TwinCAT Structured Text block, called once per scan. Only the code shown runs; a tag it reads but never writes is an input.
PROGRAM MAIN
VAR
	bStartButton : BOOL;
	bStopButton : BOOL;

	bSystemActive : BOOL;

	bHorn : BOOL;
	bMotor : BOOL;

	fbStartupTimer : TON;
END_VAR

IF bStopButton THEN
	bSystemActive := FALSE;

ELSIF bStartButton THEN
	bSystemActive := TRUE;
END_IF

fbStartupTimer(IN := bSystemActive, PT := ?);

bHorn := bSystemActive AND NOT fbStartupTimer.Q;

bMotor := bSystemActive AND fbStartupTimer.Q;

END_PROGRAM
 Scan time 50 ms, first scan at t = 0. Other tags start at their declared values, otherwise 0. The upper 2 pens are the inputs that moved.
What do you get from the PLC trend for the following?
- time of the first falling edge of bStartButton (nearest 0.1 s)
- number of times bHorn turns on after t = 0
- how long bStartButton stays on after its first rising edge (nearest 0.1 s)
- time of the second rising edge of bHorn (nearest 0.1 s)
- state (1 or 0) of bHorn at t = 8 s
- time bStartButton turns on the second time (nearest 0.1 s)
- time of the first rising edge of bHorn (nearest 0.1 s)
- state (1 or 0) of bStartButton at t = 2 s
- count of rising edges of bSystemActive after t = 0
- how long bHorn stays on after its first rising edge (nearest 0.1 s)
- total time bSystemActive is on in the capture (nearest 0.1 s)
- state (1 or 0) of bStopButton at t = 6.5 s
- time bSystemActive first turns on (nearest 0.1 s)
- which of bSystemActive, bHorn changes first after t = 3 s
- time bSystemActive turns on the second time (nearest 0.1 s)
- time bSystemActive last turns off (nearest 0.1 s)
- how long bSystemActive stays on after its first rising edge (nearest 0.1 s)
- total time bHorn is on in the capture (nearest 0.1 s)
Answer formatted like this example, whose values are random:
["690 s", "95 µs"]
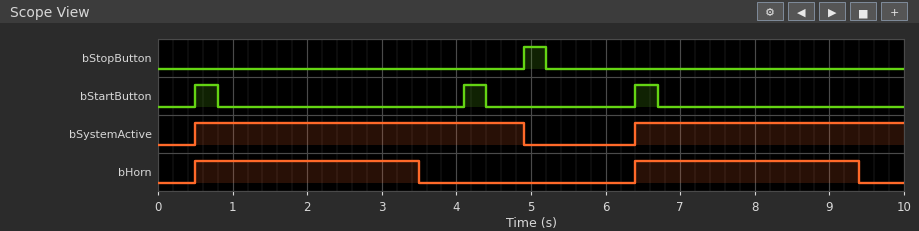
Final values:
["0.8 s", "2", "0.3 s", "6.4 s", "1", "4.1 s", "0.5 s", "0", "2", "3.0 s", "8.0 s", "0", "0.5 s", "bHorn", "6.4 s", "4.9 s", "4.4 s", "6.0 s"]
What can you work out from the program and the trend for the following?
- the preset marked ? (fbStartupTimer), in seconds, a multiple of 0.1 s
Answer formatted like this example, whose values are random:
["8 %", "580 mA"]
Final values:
["3.0 s"]
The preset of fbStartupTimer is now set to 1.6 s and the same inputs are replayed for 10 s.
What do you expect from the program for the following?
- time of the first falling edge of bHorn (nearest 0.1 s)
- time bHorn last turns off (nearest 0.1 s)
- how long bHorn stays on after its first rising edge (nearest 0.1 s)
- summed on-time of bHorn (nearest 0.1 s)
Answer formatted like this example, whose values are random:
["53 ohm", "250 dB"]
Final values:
["2.1 s", "8.0 s", "1.6 s", "3.2 s"]
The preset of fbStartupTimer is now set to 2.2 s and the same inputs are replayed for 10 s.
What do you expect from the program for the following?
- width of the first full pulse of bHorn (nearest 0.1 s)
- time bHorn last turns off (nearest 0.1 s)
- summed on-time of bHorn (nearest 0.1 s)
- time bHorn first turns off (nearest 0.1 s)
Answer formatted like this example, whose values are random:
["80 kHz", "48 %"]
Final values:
["2.2 s", "8.6 s", "4.4 s", "2.7 s"]
